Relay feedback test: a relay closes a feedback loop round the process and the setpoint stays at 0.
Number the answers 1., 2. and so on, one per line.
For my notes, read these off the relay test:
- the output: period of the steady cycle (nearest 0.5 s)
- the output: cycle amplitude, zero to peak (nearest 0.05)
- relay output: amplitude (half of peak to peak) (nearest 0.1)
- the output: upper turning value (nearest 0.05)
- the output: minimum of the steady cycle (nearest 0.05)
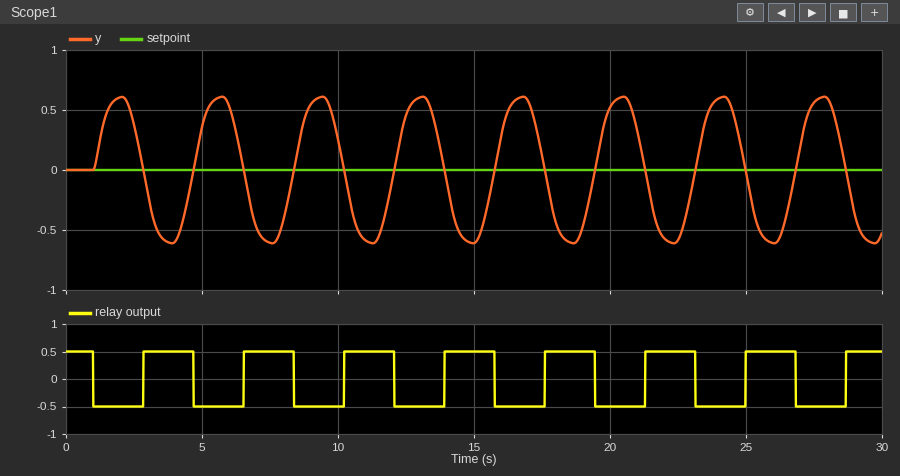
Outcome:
1. 3.5 s
2. 0.60
3. 0.5
4. 0.60
5. -0.60
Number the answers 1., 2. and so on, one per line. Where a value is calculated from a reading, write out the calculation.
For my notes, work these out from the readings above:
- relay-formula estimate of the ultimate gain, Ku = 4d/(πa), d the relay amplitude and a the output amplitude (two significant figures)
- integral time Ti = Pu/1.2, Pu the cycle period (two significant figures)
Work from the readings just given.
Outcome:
1. 4 × 0.5 / (π × 0.6) = 1.1
2. 3.5 / 1.2 = 2.9 s
